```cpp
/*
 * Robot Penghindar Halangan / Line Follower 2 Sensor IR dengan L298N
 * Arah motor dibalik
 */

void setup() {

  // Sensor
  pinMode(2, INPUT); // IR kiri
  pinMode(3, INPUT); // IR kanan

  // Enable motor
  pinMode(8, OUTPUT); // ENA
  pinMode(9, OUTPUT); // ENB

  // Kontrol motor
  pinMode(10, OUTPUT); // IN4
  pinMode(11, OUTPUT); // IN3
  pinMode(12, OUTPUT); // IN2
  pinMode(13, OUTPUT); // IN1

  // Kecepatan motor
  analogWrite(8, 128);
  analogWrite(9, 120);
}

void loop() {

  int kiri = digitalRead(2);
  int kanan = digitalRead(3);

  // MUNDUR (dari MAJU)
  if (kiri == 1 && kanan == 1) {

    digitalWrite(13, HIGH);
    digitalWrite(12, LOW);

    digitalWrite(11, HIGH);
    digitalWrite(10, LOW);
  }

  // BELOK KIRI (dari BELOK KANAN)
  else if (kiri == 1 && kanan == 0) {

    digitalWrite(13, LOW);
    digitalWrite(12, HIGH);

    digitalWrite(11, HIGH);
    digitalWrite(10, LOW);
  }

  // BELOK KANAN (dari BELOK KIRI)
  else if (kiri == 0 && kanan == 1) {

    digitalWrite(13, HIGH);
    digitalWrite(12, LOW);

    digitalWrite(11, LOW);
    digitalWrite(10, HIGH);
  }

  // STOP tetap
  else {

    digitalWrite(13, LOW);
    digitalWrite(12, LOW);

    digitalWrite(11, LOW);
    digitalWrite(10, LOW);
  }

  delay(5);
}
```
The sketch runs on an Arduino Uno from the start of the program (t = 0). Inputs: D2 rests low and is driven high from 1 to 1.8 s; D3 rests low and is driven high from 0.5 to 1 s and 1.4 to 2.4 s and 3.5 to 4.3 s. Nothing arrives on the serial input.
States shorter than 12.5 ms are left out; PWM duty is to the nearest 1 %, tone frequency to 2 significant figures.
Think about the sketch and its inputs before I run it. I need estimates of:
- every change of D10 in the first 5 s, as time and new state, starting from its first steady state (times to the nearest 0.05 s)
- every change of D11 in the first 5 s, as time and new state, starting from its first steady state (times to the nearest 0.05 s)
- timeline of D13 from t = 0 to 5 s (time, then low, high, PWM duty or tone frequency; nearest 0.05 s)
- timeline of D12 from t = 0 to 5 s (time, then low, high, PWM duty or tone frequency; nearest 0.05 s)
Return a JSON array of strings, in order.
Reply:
["0 s low; 0.5 s high; 1 s low; 1.8 s high; 2.4 s low; 3.5 s high; 4.3 s low", "0 s low; 1 s high; 1.8 s low", "0 s low; 0.5 s high; 1 s low; 1.4 s high; 2.4 s low; 3.5 s high; 4.3 s low", "0 s low; 1 s high; 1.4 s low"]
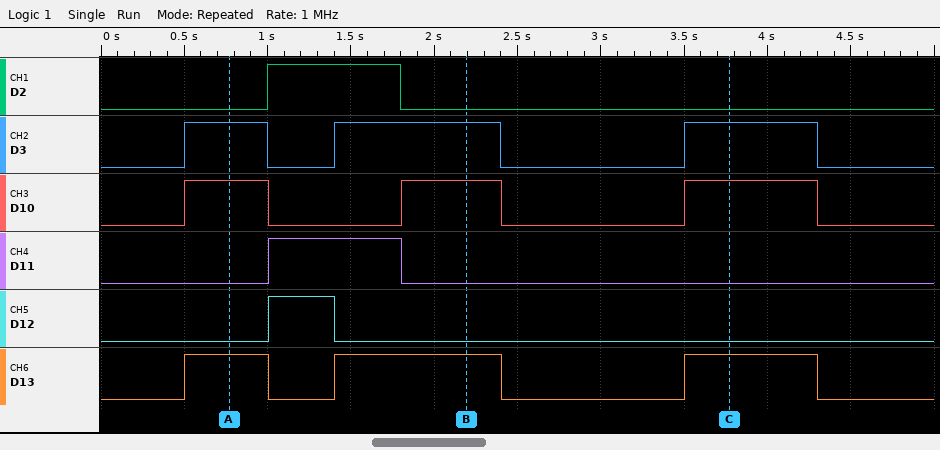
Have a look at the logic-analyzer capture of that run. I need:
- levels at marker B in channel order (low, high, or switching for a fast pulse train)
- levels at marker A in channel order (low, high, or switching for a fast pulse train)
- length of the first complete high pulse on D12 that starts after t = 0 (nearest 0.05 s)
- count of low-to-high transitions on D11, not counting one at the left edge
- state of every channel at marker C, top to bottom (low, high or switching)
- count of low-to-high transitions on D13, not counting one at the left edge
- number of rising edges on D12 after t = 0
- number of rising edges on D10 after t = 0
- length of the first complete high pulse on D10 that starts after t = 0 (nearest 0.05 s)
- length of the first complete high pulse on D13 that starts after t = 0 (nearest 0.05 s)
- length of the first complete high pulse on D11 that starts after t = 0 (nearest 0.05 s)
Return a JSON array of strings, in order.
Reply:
["D2 low, D3 high, D10 high, D11 low, D12 low, D13 high", "D2 low, D3 high, D10 high, D11 low, D12 low, D13 high", "0.40 s", "1", "D2 low, D3 high, D10 high, D11 low, D12 low, D13 high", "3", "1", "3", "0.50 s", "0.50 s", "0.80 s"]
